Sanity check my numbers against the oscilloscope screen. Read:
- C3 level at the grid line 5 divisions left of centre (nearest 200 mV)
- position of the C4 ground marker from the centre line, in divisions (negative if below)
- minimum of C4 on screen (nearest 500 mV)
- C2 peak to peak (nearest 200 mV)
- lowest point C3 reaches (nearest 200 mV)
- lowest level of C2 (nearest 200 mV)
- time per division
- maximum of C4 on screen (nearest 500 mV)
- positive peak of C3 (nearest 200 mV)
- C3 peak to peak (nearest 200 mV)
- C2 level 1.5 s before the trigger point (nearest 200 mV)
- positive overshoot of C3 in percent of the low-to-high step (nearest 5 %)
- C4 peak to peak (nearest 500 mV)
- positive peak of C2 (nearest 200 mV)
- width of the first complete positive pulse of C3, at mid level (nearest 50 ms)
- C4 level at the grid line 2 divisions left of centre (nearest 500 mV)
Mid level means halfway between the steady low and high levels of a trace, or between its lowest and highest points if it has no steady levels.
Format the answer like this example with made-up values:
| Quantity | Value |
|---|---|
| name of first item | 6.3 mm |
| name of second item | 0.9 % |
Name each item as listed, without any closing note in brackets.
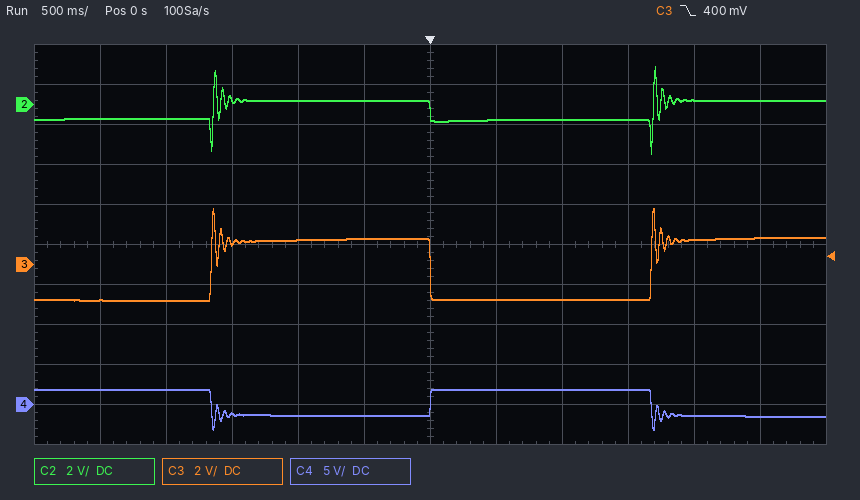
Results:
| Quantity | Value |
|---|---|
| C3 level at the grid line 5 divisions left of centre | -1.8 V |
| position of the C4 ground marker from the centre line, in divisions | -4.0 div |
| minimum of C4 on screen | -3.0 V |
| C2 peak to peak | 4.4 V |
| lowest point C3 reaches | -1.8 V |
| lowest level of C2 | -2.4 V |
| time per division | 500 ms |
| maximum of C4 on screen | 2.0 V |
| positive peak of C3 | 2.8 V |
| C3 peak to peak | 4.6 V |
| C2 level 1.5 s before the trigger point | 200 mV |
| positive overshoot of C3 in percent of the low-to-high step | 50 % |
| C4 peak to peak | 5.0 V |
| positive peak of C2 | 2.0 V |
| width of the first complete positive pulse of C3, at mid level | 1.65 s |
| C4 level at the grid line 2 divisions left of centre | -1.5 V |
